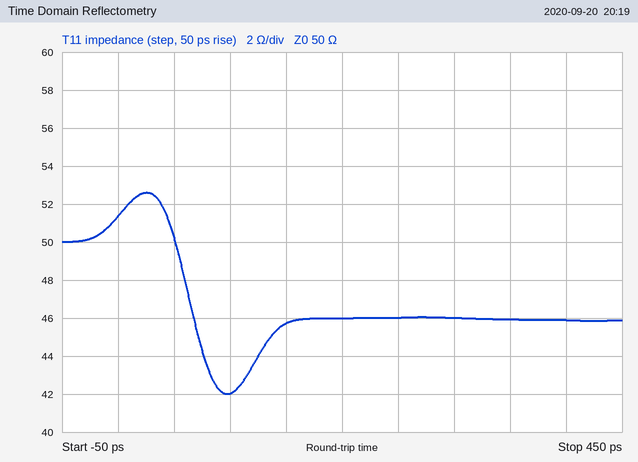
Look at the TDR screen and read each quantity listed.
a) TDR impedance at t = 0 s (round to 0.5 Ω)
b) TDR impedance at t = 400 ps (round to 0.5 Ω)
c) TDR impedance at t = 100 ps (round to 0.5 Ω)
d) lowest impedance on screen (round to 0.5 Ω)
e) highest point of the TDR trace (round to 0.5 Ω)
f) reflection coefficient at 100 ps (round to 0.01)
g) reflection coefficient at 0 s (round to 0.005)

51.5 Ω
46.0 Ω
42.0 Ω
42.0 Ω
52.5 Ω
-0.09
+0.015
